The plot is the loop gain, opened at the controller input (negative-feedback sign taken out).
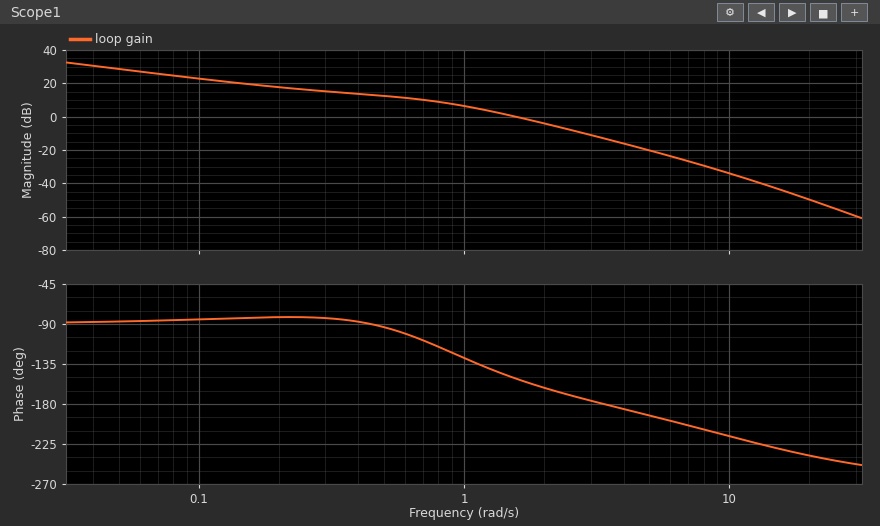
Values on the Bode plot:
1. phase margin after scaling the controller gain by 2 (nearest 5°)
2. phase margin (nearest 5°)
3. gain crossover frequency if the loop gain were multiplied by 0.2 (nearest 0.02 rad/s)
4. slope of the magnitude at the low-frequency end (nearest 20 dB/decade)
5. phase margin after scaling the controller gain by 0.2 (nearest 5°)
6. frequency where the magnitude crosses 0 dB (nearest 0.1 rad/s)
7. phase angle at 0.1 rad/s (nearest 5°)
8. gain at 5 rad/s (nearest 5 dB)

15°
30°
0.38 rad/s
-20 dB/decade
95°
1.6 rad/s
-85°
-20 dB
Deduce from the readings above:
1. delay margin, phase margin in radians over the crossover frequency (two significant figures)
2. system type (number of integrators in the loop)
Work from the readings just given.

0.33 s
1
